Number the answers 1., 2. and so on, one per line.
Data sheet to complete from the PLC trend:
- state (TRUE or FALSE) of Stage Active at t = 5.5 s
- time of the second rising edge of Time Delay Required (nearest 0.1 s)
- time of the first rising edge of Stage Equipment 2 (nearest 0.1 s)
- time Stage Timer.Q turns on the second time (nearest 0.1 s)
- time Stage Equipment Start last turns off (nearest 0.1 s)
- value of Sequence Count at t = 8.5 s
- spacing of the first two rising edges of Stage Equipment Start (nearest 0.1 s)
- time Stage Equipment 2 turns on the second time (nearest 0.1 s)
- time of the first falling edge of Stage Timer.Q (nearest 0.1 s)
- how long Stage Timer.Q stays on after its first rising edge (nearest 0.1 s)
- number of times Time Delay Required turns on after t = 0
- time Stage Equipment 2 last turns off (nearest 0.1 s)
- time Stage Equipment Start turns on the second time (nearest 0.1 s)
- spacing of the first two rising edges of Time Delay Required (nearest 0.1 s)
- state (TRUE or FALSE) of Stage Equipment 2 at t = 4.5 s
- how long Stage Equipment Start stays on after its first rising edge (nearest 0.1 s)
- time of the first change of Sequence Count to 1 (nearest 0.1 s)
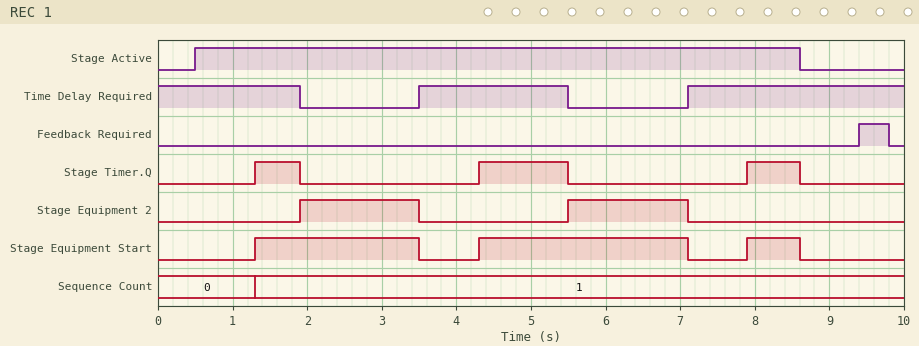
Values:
1. TRUE
2. 7.1 s
3. 1.9 s
4. 4.3 s
5. 8.6 s
6. 1
7. 3.0 s
8. 5.5 s
9. 1.9 s
10. 0.6 s
11. 2
12. 7.1 s
13. 4.3 s
14. 3.6 s
15. FALSE
16. 2.2 s
17. 1.3 s
